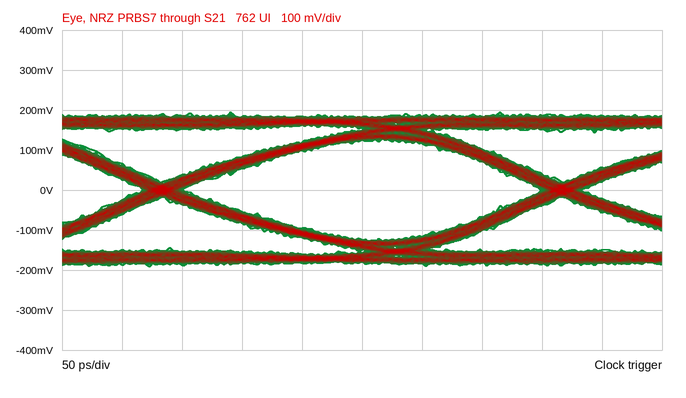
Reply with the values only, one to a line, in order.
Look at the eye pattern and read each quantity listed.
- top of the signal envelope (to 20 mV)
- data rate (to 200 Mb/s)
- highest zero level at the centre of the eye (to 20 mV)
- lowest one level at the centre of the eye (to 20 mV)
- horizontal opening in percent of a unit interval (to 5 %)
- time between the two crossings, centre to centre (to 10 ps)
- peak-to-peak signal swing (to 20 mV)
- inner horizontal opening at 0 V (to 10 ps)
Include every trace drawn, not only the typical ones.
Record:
200 mV
3.0 Gb/s
-120 mV
120 mV
90 %
330 ps
380 mV
300 ps
